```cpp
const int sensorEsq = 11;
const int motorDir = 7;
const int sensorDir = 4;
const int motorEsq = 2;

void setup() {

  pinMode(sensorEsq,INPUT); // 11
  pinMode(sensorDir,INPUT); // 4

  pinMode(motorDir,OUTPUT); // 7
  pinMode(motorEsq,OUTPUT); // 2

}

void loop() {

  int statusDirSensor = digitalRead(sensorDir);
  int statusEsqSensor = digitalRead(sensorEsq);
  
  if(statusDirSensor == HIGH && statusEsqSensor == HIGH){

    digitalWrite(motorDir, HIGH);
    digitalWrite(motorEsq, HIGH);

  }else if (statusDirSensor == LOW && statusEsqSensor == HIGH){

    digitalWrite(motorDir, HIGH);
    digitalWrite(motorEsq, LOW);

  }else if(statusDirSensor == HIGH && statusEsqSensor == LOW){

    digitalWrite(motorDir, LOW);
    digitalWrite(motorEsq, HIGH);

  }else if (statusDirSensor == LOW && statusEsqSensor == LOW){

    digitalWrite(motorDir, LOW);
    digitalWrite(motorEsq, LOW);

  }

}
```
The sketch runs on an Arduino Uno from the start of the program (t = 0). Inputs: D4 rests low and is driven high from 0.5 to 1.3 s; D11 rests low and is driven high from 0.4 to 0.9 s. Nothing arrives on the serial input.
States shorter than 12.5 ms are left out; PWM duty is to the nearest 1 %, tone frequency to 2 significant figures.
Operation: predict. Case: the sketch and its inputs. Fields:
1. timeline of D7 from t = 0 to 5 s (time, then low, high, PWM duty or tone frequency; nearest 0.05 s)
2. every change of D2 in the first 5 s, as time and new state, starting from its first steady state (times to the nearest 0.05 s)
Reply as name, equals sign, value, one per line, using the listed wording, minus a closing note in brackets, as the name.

timeline of D7 from t = 0 to 5 s = 0 s low; 0.4 s high; 0.9 s low
every change of D2 in the first 5 s, as time and new state, starting from its first steady state = 0 s low; 0.5 s high; 1.3 s low
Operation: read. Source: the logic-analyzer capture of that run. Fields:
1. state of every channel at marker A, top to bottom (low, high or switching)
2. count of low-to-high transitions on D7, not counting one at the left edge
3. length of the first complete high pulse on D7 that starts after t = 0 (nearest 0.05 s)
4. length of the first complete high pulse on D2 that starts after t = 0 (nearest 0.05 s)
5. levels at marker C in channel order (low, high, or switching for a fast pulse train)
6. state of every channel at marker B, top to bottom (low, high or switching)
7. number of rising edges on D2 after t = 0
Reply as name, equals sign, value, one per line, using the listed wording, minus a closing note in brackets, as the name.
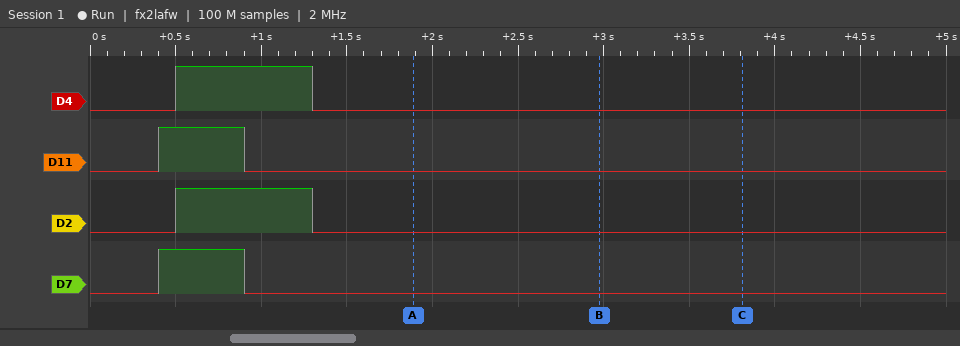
state of every channel at marker A, top to bottom = D4 low, D11 low, D2 low, D7 low
count of low-to-high transitions on D7, not counting one at the left edge = 1
length of the first complete high pulse on D7 that starts after t = 0 = 0.50 s
length of the first complete high pulse on D2 that starts after t = 0 = 0.80 s
levels at marker C in channel order = D4 low, D11 low, D2 low, D7 low
state of every channel at marker B, top to bottom = D4 low, D11 low, D2 low, D7 low
number of rising edges on D2 after t = 0 = 1
